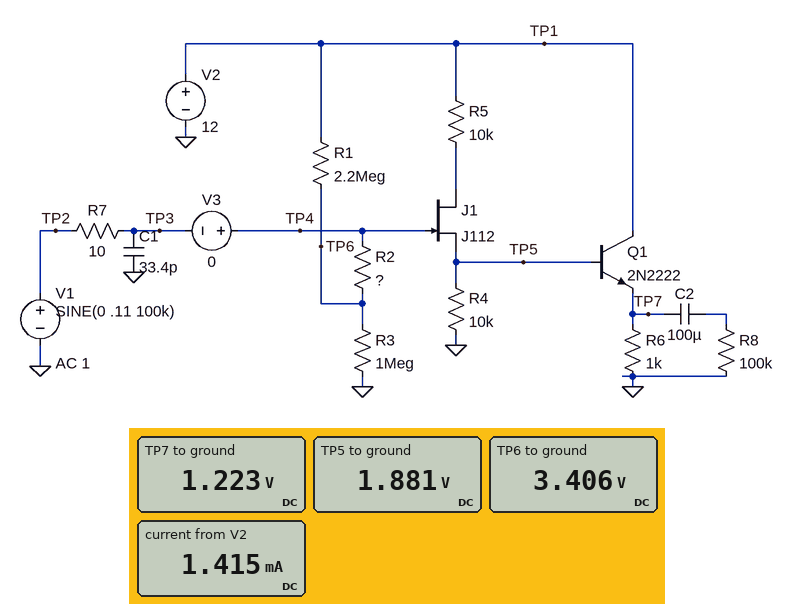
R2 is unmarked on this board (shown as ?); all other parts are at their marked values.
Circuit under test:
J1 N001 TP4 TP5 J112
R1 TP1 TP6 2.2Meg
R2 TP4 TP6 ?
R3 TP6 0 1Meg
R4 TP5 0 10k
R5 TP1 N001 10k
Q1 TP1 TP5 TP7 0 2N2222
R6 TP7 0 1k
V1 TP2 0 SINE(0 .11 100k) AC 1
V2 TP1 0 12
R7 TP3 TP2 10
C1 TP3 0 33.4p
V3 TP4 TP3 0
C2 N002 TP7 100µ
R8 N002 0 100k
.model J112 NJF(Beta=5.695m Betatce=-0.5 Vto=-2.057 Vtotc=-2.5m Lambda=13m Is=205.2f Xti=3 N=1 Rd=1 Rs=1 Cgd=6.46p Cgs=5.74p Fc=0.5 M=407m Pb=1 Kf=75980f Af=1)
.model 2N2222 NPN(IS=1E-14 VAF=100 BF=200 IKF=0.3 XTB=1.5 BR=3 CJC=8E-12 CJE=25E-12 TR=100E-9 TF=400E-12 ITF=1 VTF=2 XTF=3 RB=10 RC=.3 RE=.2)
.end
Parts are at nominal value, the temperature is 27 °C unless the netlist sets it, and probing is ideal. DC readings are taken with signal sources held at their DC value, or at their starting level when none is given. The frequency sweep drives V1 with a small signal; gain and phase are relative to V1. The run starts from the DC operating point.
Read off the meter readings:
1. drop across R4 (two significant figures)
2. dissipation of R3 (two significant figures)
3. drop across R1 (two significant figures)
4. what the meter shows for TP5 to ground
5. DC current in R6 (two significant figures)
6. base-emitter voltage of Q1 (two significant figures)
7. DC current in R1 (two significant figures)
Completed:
1.9 V
12 µW
8.6 V
1.881 V
1.2 mA
660 mV
3.9 µA
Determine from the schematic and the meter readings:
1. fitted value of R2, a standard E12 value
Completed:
6.8 MΩ
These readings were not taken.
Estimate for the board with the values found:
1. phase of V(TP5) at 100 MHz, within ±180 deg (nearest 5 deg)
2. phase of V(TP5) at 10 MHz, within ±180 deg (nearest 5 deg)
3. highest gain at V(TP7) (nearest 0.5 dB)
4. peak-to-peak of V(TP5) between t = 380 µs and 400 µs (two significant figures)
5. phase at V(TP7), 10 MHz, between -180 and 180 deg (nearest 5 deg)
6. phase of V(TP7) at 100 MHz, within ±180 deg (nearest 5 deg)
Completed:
-30 deg
-10 deg
-0.5 dB
210 mV
-10 deg
-30 deg
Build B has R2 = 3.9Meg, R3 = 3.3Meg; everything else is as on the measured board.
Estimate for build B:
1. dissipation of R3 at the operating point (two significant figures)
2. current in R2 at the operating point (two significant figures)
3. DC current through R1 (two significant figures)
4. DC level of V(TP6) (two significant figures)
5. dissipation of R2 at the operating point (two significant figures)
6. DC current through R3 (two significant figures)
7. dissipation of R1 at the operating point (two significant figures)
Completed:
8.8 µW
1.4 µA
3.0 µA
5.4 V
7.4 µW
1.6 µA
20 µW
